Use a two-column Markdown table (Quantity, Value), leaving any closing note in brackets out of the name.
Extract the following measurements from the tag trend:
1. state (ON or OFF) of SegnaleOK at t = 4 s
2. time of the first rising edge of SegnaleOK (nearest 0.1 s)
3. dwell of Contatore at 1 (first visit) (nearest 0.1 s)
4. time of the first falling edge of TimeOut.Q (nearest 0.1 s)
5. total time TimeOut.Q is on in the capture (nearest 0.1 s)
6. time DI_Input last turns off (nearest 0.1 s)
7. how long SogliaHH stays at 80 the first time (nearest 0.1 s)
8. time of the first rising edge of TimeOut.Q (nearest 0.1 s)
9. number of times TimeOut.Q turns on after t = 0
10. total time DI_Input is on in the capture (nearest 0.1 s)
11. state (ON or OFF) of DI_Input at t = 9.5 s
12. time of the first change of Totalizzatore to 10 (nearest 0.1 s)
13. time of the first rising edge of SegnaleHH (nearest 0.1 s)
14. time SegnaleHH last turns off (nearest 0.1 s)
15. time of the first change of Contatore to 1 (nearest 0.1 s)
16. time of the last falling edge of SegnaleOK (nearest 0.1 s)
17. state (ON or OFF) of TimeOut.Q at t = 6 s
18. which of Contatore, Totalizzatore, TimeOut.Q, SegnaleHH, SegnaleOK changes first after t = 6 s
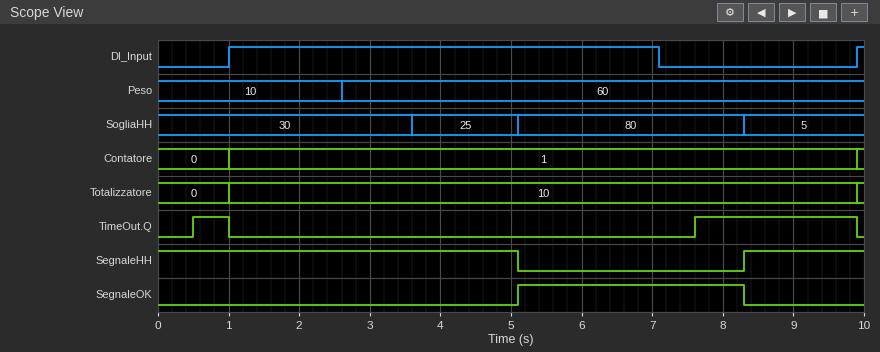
| Quantity | Value |
|---|---|
| state (ON or OFF) of SegnaleOK at t = 4 s | OFF |
| time of the first rising edge of SegnaleOK | 5.1 s |
| dwell of Contatore at 1 (first visit) | 8.9 s |
| time of the first falling edge of TimeOut.Q | 1.0 s |
| total time TimeOut.Q is on in the capture | 2.8 s |
| time DI_Input last turns off | 7.1 s |
| how long SogliaHH stays at 80 the first time | 3.2 s |
| time of the first rising edge of TimeOut.Q | 0.5 s |
| number of times TimeOut.Q turns on after t = 0 | 2 |
| total time DI_Input is on in the capture | 6.2 s |
| state (ON or OFF) of DI_Input at t = 9.5 s | OFF |
| time of the first change of Totalizzatore to 10 | 1.0 s |
| time of the first rising edge of SegnaleHH | 8.3 s |
| time SegnaleHH last turns off | 5.1 s |
| time of the first change of Contatore to 1 | 1.0 s |
| time of the last falling edge of SegnaleOK | 8.3 s |
| state (ON or OFF) of TimeOut.Q at t = 6 s | OFF |
| which of Contatore, Totalizzatore, TimeOut.Q, SegnaleHH, SegnaleOK changes first after t = 6 s | TimeOut.Q |
